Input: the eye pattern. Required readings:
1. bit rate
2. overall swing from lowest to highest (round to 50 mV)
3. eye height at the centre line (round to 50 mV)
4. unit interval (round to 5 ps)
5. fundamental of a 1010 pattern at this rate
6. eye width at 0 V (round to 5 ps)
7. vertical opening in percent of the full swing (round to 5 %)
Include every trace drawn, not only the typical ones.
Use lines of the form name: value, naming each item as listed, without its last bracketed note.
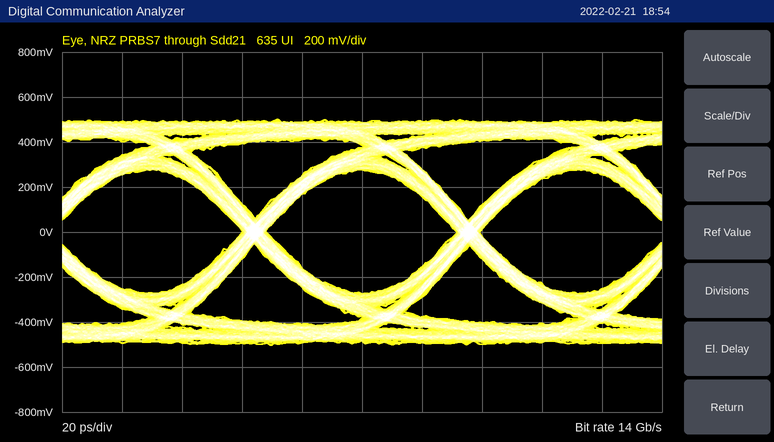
bit rate: 14 Gb/s
overall swing from lowest to highest: 1.00 V
eye height at the centre line: 550 mV
unit interval: 70 ps
fundamental of a 1010 pattern at this rate: 7 GHz
eye width at 0 V: 65 ps
vertical opening in percent of the full swing: 55 %
